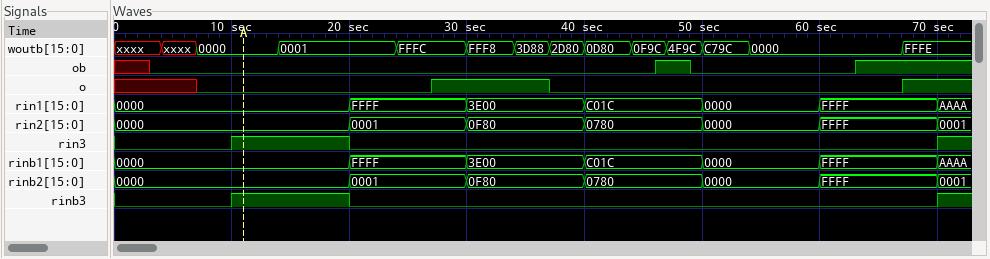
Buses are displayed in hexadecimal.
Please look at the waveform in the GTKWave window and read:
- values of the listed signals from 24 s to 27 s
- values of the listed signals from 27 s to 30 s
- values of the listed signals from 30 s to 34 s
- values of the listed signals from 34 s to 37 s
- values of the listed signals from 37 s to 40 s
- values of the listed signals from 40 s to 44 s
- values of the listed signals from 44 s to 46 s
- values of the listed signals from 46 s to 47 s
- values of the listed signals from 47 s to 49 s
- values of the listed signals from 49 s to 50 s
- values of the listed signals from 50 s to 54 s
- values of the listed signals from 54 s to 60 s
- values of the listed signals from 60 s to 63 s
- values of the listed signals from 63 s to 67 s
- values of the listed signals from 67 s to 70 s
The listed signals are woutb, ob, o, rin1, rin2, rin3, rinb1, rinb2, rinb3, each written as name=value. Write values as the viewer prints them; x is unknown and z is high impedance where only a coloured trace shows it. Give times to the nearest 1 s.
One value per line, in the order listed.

woutb=FFFC, ob=0, o=0, rin1=FFFF, rin2=0001, rin3=0, rinb1=FFFF, rinb2=0001, rinb3=0
woutb=FFFC, ob=0, o=1, rin1=FFFF, rin2=0001, rin3=0, rinb1=FFFF, rinb2=0001, rinb3=0
woutb=FFF8, ob=0, o=1, rin1=3E00, rin2=0F80, rin3=0, rinb1=3E00, rinb2=0F80, rinb3=0
woutb=3D88, ob=0, o=1, rin1=3E00, rin2=0F80, rin3=0, rinb1=3E00, rinb2=0F80, rinb3=0
woutb=2D80, ob=0, o=0, rin1=3E00, rin2=0F80, rin3=0, rinb1=3E00, rinb2=0F80, rinb3=0
woutb=0D80, ob=0, o=0, rin1=C01C, rin2=0780, rin3=0, rinb1=C01C, rinb2=0780, rinb3=0
woutb=0F9C, ob=0, o=0, rin1=C01C, rin2=0780, rin3=0, rinb1=C01C, rinb2=0780, rinb3=0
woutb=0F9C, ob=1, o=0, rin1=C01C, rin2=0780, rin3=0, rinb1=C01C, rinb2=0780, rinb3=0
woutb=4F9C, ob=1, o=0, rin1=C01C, rin2=0780, rin3=0, rinb1=C01C, rinb2=0780, rinb3=0
woutb=4F9C, ob=0, o=0, rin1=C01C, rin2=0780, rin3=0, rinb1=C01C, rinb2=0780, rinb3=0
woutb=C79C, ob=0, o=0, rin1=0000, rin2=0000, rin3=0, rinb1=0000, rinb2=0000, rinb3=0
woutb=0000, ob=0, o=0, rin1=0000, rin2=0000, rin3=0, rinb1=0000, rinb2=0000, rinb3=0
woutb=0000, ob=0, o=0, rin1=FFFF, rin2=FFFF, rin3=0, rinb1=FFFF, rinb2=FFFF, rinb3=0
woutb=0000, ob=1, o=0, rin1=FFFF, rin2=FFFF, rin3=0, rinb1=FFFF, rinb2=FFFF, rinb3=0
woutb=FFFE, ob=1, o=1, rin1=FFFF, rin2=FFFF, rin3=0, rinb1=FFFF, rinb2=FFFF, rinb3=0
